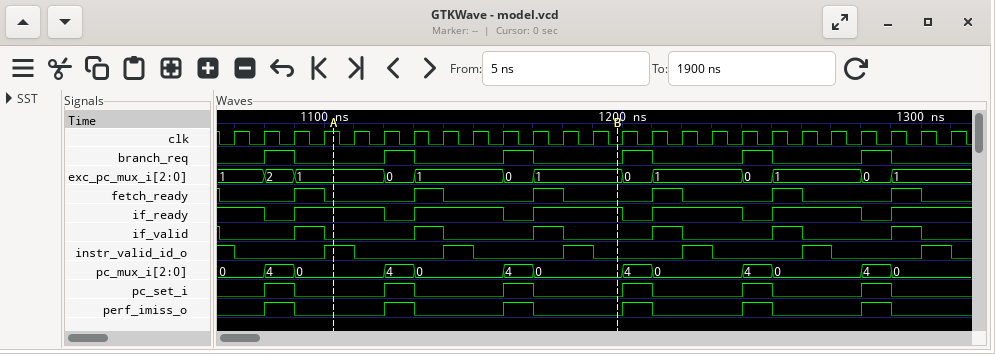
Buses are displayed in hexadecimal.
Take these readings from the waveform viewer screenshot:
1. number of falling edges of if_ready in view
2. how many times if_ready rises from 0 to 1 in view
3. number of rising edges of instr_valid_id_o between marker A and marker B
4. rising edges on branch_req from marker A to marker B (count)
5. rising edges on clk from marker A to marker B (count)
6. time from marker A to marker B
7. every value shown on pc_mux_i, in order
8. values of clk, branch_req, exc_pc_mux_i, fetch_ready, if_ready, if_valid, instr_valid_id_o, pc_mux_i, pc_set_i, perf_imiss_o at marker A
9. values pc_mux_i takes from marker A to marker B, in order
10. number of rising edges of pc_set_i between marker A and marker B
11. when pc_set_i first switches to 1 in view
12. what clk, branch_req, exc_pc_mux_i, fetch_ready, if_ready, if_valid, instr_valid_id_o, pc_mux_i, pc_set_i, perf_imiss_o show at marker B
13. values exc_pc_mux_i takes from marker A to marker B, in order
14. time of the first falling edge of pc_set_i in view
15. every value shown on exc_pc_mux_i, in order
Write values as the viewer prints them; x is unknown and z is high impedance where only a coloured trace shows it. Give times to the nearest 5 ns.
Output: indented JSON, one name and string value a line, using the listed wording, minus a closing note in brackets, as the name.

{
  "number of falling edges of if_ready in view": "6",
  "how many times if_ready rises from 0 to 1 in view": "6",
  "number of rising edges of instr_valid_id_o between marker A and marker B": "2",
  "rising edges on branch_req from marker A to marker B": "2",
  "rising edges on clk from marker A to marker B": "9",
  "time from marker A to marker B": "95 ns",
  "every value shown on pc_mux_i, in order": "0, 4, 0, 4, 0, 4, 0, 4, 0, 4, 0, 4, 0",
  "values of clk, branch_req, exc_pc_mux_i, fetch_ready, if_ready, if_valid, instr_valid_id_o, pc_mux_i, pc_set_i, perf_imiss_o at marker A": "clk=1, branch_req=0, exc_pc_mux_i=1, fetch_ready=0, if_ready=1, if_valid=0, instr_valid_id_o=1, pc_mux_i=0, pc_set_i=0, perf_imiss_o=0",
  "values pc_mux_i takes from marker A to marker B, in order": "0, 4, 0, 4, 0",
  "number of rising edges of pc_set_i between marker A and marker B": "2",
  "when pc_set_i first switches to 1 in view": "1080 ns",
  "what clk, branch_req, exc_pc_mux_i, fetch_ready, if_ready, if_valid, instr_valid_id_o, pc_mux_i, pc_set_i, perf_imiss_o show at marker B": "clk=0, branch_req=0, exc_pc_mux_i=1, fetch_ready=0, if_ready=1, if_valid=0, instr_valid_id_o=0, pc_mux_i=0, pc_set_i=0, perf_imiss_o=0",
  "values exc_pc_mux_i takes from marker A to marker B, in order": "1, 0, 1, 0, 1",
  "time of the first falling edge of pc_set_i in view": "1090 ns",
  "every value shown on exc_pc_mux_i, in order": "1, 2, 1, 0, 1, 0, 1, 0, 1, 0, 1, 0, 1"
}
